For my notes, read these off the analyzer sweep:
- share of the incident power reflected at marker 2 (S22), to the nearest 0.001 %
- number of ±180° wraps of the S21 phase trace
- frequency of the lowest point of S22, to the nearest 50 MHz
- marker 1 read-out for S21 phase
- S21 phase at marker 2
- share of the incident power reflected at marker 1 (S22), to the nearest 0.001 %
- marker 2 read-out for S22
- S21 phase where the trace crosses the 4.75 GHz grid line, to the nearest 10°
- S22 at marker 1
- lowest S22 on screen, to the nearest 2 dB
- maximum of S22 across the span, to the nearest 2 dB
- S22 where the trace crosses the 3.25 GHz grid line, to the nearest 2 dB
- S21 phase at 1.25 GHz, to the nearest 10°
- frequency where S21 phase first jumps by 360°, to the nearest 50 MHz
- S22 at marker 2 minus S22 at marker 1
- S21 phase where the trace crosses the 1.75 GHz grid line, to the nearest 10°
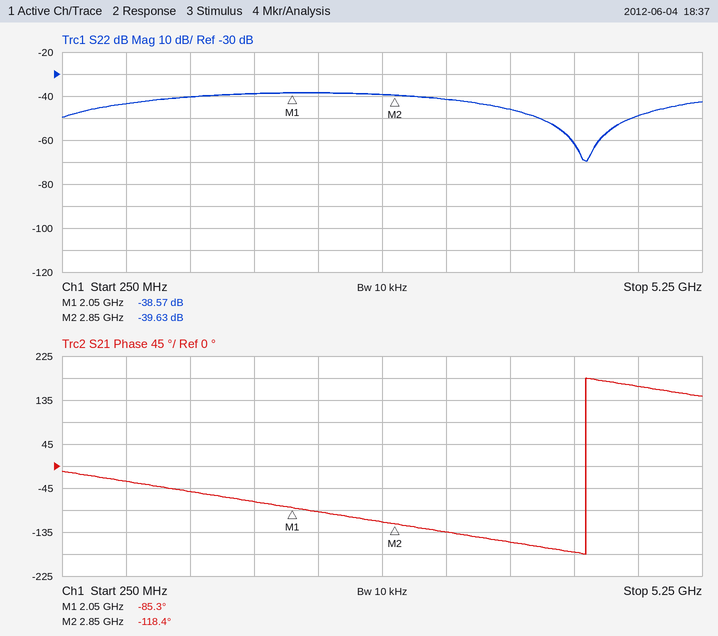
0.011 %
1
4.35 GHz
-85.3°
-118.4°
0.014 %
-39.63 dB
160°
-38.57 dB
-70 dB
-38 dB
-42 dB
-50°
4.35 GHz
-1.06 dB
-70°
